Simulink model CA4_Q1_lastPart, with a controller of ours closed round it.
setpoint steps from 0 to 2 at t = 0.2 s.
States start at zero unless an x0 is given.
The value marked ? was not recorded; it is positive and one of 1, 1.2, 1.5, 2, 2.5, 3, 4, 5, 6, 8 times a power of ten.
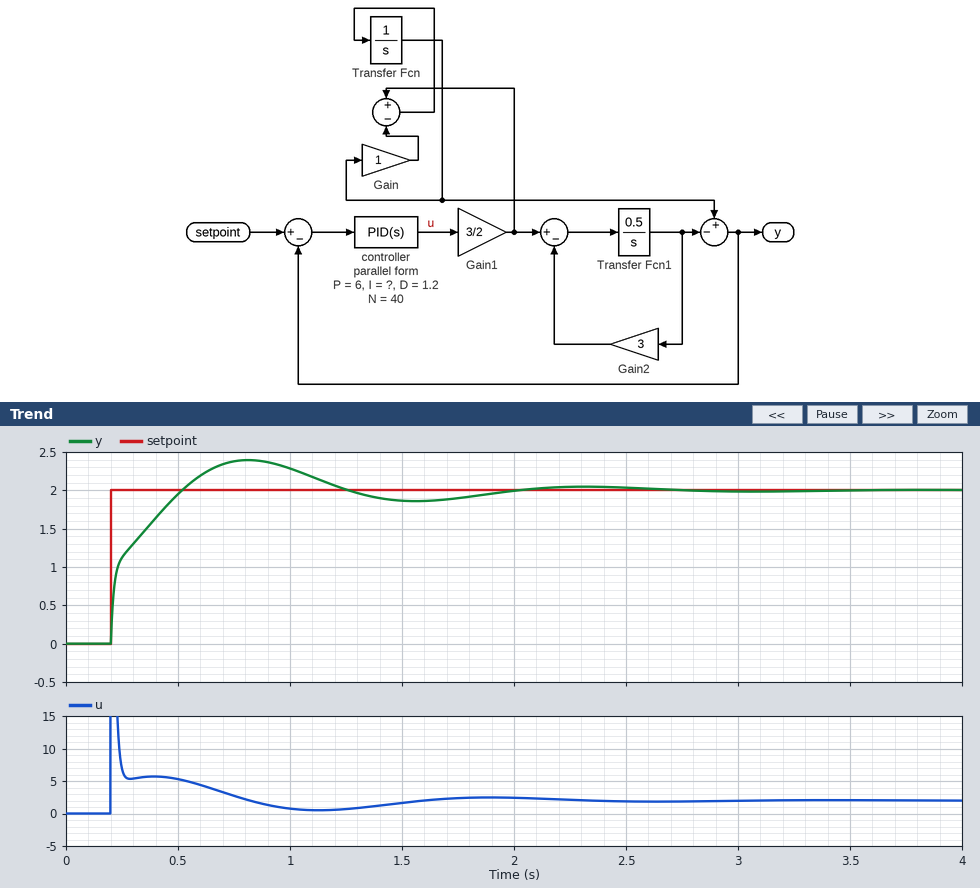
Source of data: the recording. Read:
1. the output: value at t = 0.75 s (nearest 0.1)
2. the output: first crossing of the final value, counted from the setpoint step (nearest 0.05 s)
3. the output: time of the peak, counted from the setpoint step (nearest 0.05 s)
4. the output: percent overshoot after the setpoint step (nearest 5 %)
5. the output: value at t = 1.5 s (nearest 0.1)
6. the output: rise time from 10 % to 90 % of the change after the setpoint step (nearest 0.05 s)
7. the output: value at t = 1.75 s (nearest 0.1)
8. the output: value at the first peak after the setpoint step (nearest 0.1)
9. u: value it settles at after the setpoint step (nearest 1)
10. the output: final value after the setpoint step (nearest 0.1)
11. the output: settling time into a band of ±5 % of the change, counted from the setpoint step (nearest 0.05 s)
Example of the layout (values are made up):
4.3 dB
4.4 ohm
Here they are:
2.4
0.30 s
0.60 s
20 %
1.9
0.25 s
1.9
2.4
2
2.0
1.55 s
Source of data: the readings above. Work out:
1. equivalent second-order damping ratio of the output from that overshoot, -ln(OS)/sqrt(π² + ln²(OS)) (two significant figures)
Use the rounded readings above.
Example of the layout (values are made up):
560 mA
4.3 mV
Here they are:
0.46
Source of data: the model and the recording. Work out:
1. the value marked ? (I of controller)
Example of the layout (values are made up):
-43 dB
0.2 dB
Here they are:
50
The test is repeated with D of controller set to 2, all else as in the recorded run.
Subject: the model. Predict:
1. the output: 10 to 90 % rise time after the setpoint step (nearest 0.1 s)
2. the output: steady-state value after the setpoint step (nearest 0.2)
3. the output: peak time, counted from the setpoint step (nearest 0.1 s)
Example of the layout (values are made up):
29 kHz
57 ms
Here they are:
0.3 s
2.0
0.7 s
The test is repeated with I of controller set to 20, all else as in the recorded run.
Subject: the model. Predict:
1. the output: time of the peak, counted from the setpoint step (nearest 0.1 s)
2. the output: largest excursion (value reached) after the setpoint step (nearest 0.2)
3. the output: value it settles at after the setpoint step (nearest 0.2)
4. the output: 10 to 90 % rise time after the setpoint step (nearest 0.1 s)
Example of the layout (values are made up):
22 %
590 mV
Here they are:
0.9 s
2.2
2.0
0.4 s
